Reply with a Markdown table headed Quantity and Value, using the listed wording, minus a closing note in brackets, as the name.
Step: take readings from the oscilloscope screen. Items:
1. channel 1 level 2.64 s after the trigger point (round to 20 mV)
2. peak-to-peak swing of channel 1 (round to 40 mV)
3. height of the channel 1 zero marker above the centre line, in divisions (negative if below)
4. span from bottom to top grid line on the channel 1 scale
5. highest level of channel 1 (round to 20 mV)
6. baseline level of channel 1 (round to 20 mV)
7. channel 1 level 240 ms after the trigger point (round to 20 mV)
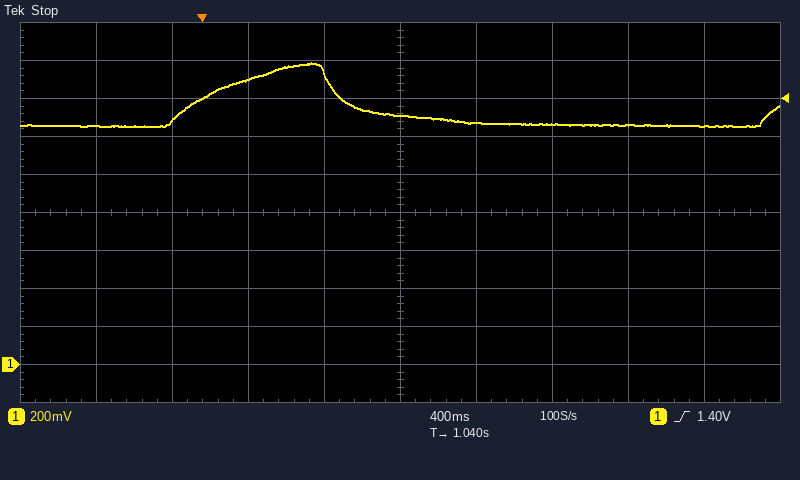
| Quantity | Value |
|---|---|
| channel 1 level 2.64 s after the trigger point | 1.26 V |
| peak-to-peak swing of channel 1 | 320 mV |
| height of the channel 1 zero marker above the centre line, in divisions | -4.0 div |
| span from bottom to top grid line on the channel 1 scale | 2 V |
| highest level of channel 1 | 1.58 V |
| baseline level of channel 1 | 1.26 V |
| channel 1 level 240 ms after the trigger point | 1.50 V |
